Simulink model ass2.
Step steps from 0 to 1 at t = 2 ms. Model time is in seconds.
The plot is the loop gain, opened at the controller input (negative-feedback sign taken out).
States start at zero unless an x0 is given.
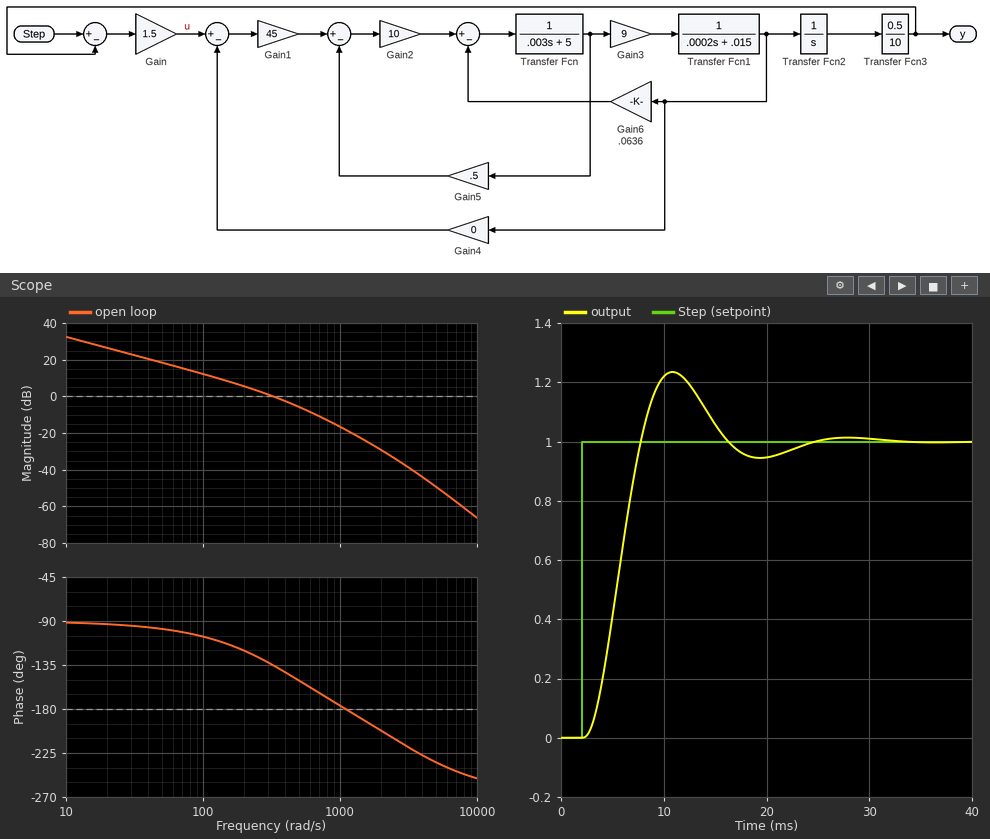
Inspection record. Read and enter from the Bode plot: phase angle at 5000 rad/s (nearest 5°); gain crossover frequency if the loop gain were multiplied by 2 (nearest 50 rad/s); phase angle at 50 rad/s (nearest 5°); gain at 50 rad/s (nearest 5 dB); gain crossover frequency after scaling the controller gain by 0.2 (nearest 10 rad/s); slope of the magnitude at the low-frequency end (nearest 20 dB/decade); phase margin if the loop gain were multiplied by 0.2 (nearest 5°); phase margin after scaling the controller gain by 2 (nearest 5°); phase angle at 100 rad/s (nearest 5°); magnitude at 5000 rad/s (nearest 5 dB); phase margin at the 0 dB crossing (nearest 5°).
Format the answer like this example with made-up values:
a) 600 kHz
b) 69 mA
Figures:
a) -235°
b) 500 rad/s
c) -100°
d) 20 dB
e) 80 rad/s
f) -20 dB/decade
g) 75°
h) 30°
i) -105°
j) -50 dB
k) 45°
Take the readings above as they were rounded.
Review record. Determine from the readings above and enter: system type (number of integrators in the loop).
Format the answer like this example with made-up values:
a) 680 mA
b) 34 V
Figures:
a) 1
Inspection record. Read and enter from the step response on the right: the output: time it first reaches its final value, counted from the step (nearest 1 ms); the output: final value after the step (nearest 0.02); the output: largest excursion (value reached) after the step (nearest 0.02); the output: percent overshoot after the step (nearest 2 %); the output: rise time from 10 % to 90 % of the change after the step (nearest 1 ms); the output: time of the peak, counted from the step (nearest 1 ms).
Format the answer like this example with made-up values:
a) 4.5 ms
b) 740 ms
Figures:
a) 6 ms
b) 1.00
c) 1.24
d) 24 %
e) 4 ms
f) 9 ms
